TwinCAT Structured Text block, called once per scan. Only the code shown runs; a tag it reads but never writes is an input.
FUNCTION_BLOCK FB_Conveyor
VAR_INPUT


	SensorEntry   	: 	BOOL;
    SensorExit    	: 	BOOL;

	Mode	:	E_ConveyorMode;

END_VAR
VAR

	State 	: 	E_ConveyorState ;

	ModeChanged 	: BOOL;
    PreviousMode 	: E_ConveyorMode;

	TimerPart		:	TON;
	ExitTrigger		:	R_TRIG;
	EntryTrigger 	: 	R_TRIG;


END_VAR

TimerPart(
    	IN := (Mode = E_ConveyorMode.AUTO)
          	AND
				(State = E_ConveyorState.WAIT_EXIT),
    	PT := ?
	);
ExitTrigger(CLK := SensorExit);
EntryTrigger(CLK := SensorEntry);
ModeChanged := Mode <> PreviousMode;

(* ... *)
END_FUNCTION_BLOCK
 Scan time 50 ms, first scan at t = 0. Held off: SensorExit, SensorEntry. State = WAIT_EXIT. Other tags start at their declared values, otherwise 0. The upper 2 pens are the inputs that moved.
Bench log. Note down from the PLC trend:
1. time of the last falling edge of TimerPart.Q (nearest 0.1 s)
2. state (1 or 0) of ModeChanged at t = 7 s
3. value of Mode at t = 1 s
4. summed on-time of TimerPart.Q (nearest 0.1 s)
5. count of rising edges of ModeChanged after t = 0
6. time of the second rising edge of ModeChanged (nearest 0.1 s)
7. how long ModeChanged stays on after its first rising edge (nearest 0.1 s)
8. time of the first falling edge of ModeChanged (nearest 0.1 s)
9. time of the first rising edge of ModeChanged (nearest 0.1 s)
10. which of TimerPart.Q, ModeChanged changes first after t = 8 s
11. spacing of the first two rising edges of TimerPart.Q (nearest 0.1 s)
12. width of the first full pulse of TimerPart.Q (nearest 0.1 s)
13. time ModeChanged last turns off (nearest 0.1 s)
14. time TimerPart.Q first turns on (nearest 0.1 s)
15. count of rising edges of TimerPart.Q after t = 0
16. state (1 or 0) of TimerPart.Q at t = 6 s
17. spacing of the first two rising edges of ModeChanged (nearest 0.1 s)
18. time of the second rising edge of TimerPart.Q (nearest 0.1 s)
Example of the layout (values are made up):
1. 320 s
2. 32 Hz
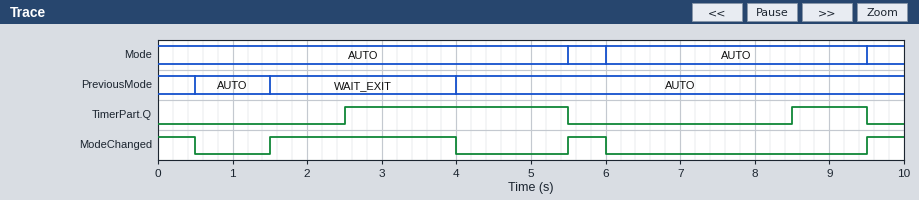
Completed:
1. 9.5 s
2. 0
3. AUTO
4. 4.0 s
5. 3
6. 5.5 s
7. 2.5 s
8. 0.5 s
9. 1.5 s
10. TimerPart.Q
11. 6.0 s
12. 3.0 s
13. 6.0 s
14. 2.5 s
15. 2
16. 0
17. 4.0 s
18. 8.5 s
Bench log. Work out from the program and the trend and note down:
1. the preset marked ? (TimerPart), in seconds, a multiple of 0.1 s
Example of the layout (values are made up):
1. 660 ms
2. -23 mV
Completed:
1. 2.5 s
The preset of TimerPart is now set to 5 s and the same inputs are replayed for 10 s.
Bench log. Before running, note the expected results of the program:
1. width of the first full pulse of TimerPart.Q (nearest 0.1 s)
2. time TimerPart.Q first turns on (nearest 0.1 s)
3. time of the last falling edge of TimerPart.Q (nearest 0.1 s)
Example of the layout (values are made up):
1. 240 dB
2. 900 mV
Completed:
1. 0.5 s
2. 5.0 s
3. 5.5 s
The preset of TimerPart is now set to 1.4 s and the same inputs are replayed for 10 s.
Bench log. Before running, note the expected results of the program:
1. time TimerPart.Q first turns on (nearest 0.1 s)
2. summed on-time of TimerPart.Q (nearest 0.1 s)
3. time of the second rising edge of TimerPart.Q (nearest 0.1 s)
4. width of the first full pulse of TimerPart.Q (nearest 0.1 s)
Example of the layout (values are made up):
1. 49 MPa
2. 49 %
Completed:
1. 1.4 s
2. 6.2 s
3. 7.4 s
4. 4.1 s
